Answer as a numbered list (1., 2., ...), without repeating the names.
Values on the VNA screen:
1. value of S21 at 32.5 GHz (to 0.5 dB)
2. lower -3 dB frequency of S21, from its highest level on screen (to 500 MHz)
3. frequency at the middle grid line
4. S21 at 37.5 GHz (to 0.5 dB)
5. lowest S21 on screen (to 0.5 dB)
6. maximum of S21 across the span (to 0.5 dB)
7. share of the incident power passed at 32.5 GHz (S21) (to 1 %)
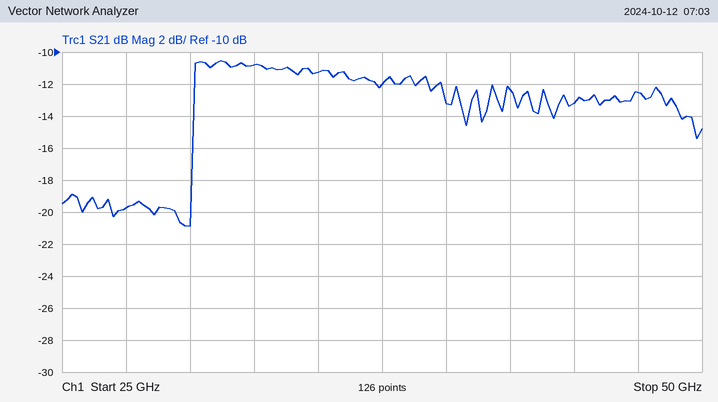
1. -11.0 dB
2. 30.0 GHz
3. 37.5 GHz
4. -12.0 dB
5. -21.0 dB
6. -10.5 dB
7. 8 %
